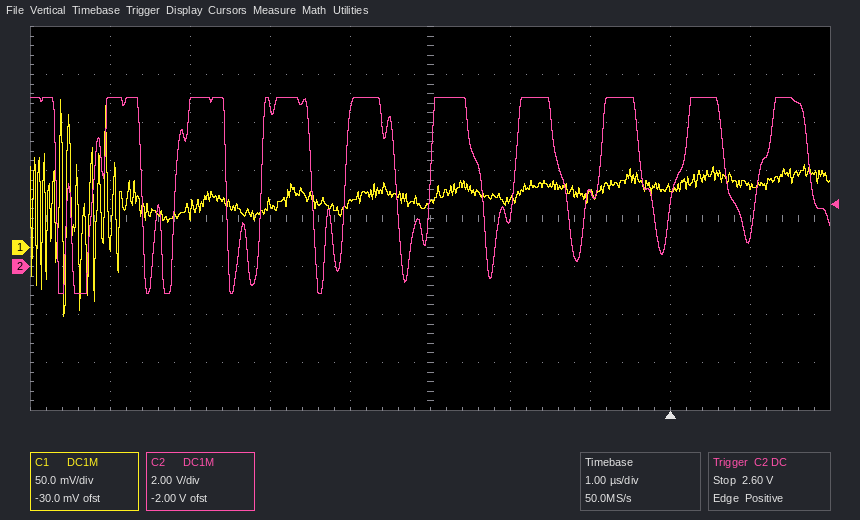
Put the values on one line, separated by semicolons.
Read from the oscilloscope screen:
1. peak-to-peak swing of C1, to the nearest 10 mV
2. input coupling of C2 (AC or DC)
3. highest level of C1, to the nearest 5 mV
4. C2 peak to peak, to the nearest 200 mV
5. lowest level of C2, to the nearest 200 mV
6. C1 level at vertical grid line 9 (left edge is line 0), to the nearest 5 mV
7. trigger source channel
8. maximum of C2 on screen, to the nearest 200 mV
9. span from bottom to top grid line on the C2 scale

230 mV; DC; 155 mV; 8.2 V; -1.2 V; 65 mV; C2; 7.0 V; 16 V
